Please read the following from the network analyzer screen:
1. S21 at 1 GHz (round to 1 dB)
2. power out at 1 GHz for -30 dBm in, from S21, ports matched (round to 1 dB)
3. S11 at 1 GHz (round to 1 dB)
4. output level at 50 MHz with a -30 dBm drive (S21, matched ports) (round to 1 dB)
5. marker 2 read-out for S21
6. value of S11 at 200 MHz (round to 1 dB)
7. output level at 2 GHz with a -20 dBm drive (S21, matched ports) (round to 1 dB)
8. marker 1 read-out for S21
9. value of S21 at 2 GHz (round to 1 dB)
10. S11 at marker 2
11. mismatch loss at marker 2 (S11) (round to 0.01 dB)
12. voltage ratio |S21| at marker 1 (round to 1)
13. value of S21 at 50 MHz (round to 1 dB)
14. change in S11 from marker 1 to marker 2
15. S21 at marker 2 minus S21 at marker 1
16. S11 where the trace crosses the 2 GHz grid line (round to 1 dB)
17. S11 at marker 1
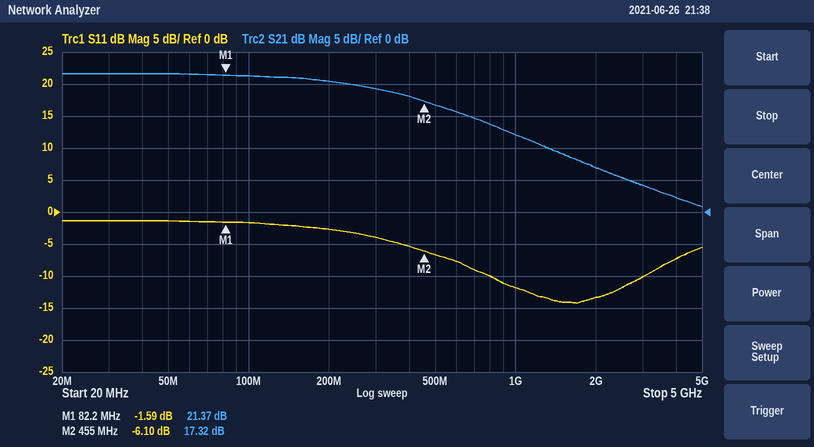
12 dB
-18 dBm
-12 dB
-8 dBm
17.32 dB
-3 dB
-13 dBm
21.37 dB
7 dB
-6.10 dB
1.22 dB
12
22 dB
-4.51 dB
-4.05 dB
-13 dB
-1.59 dB
